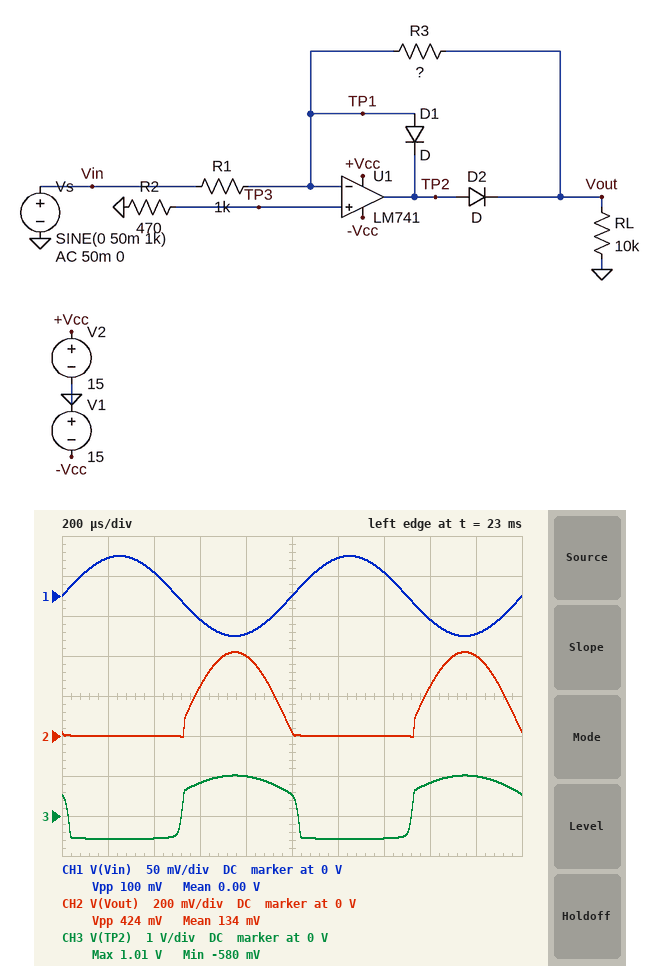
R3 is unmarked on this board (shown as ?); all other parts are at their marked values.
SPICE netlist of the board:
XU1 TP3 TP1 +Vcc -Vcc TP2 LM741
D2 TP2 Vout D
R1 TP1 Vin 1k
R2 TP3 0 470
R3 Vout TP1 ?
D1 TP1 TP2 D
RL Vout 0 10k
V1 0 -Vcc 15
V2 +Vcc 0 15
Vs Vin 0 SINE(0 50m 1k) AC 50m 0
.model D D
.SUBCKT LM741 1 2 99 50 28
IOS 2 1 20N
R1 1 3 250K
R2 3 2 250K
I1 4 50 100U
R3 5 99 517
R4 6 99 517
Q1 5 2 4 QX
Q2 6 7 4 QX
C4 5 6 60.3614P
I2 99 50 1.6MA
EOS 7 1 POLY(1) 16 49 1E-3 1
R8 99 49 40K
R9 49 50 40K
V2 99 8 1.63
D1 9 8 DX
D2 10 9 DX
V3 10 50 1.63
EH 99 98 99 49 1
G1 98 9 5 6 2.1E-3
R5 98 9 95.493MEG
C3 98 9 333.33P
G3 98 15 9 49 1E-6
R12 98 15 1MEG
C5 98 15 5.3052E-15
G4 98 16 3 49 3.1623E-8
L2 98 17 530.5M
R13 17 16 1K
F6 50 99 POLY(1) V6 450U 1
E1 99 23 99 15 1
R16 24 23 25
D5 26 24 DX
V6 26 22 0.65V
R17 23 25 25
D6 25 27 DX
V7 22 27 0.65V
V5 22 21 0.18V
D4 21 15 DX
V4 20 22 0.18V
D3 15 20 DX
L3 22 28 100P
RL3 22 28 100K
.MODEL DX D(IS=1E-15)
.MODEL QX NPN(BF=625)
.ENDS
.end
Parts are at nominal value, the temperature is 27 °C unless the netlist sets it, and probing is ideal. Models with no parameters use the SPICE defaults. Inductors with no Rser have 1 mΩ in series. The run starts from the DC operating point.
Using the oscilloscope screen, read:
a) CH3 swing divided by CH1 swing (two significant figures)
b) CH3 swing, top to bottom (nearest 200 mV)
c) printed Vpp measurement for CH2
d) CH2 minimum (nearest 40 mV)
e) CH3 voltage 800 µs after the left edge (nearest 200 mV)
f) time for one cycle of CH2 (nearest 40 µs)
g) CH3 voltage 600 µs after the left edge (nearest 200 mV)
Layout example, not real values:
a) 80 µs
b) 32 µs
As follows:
a) 16
b) 1.6 V
c) 424 mV
d) 0 V
e) 1.0 V
f) 1.00 ms
g) 800 mV
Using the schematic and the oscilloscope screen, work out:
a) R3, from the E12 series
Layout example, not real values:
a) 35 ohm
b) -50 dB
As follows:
a) 8.2 kΩ
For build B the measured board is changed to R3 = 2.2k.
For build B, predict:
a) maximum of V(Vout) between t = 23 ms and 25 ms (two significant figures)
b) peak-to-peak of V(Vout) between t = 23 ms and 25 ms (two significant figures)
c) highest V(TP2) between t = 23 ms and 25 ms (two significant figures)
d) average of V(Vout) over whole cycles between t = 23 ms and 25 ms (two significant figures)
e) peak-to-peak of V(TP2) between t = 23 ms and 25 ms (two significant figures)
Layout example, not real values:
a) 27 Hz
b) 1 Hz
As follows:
a) 110 mV
b) 120 mV
c) 700 mV
d) 37 mV
e) 1.3 V
